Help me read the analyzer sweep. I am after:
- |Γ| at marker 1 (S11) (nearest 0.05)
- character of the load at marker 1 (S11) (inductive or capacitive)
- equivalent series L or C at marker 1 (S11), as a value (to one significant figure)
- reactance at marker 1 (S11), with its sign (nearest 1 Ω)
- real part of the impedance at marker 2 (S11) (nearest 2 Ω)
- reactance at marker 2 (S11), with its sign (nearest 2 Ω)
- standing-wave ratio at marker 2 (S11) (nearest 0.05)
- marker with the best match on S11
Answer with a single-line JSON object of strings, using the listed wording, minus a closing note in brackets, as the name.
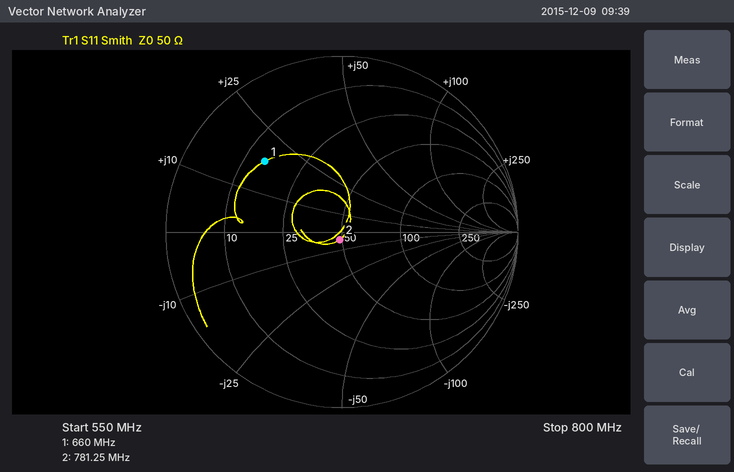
{"|Γ| at marker 1 (S11)": "0.60", "character of the load at marker 1 (S11)": "inductive", "equivalent series L or C at marker 1 (S11), as a value": "4 nH", "reactance at marker 1 (S11), with its sign": "+18 Ω", "real part of the impedance at marker 2 (S11)": "48 Ω", "reactance at marker 2 (S11), with its sign": "-4 Ω", "standing-wave ratio at marker 2 (S11)": "1.10", "marker with the best match on S11": "marker 2"}
